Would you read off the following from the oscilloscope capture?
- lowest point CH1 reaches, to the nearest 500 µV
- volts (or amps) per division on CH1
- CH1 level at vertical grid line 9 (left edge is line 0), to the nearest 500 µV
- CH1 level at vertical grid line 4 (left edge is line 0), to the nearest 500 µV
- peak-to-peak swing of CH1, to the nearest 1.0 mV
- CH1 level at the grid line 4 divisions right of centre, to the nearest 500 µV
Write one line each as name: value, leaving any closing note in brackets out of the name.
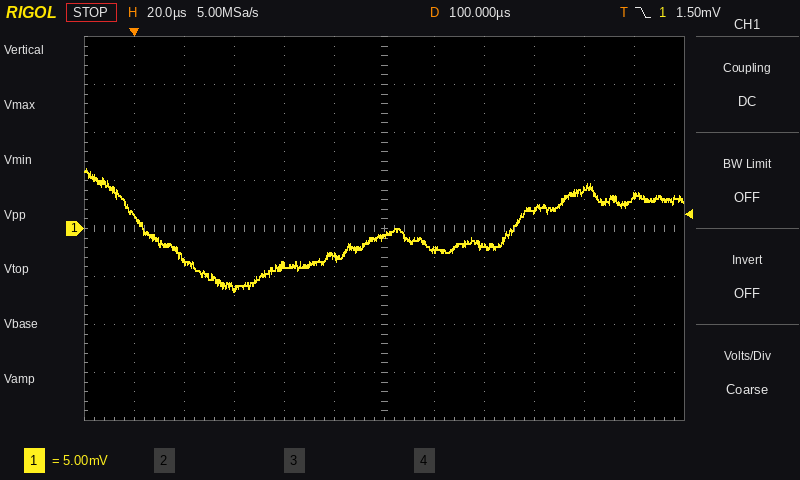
lowest point CH1 reaches, to the nearest 500 µV: -6.5 mV
volts (or amps) per division on CH1: 5 mV
CH1 level at vertical grid line 9 (left edge is line 0), to the nearest 500 µV: 2.0 mV
CH1 level at vertical grid line 4 (left edge is line 0), to the nearest 500 µV: -4.0 mV
peak-to-peak swing of CH1, to the nearest 1.0 mV: 13.0 mV
CH1 level at the grid line 4 divisions right of centre, to the nearest 500 µV: 4.0 mV
